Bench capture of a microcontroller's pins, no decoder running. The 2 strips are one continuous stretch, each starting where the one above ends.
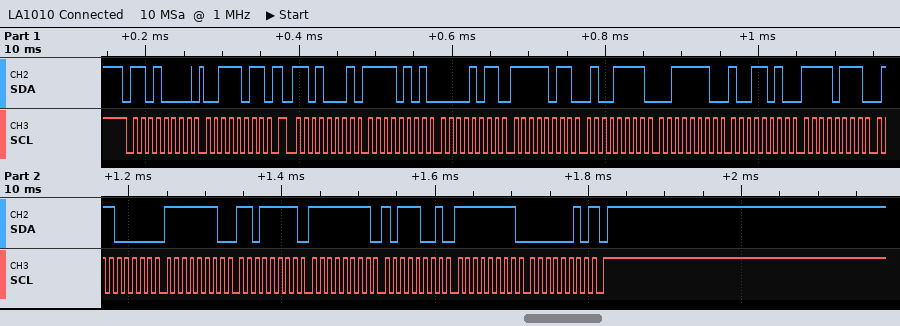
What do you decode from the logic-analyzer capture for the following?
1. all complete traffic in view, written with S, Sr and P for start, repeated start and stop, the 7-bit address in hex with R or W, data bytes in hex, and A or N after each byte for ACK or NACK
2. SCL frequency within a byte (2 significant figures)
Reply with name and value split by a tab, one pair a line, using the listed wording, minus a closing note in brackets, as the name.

all complete traffic in view, written with S, Sr and P for start, repeated start and stop, the 7-bit address in hex with R or W, data bytes in hex, and A or N after each byte for ACK or NACK	S 68W A 3B A Sr 68R A F5 A 0B A FB A 4F A 3E A 9A A F7 A 60 A FE A DF A FF A B9 A FF A 02 N P
SCL frequency within a byte	100 kHz
